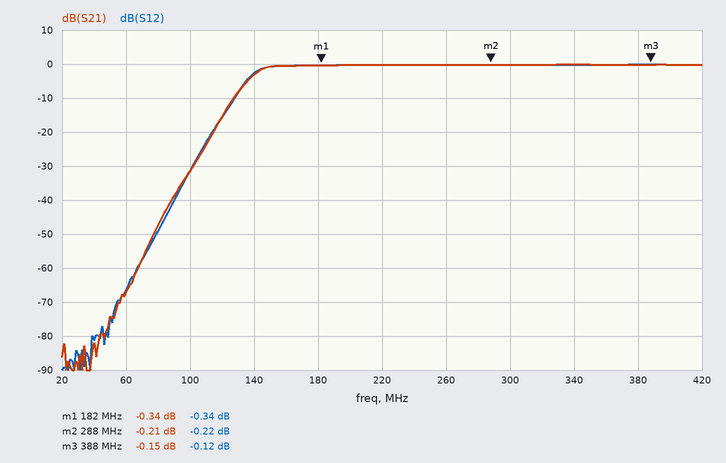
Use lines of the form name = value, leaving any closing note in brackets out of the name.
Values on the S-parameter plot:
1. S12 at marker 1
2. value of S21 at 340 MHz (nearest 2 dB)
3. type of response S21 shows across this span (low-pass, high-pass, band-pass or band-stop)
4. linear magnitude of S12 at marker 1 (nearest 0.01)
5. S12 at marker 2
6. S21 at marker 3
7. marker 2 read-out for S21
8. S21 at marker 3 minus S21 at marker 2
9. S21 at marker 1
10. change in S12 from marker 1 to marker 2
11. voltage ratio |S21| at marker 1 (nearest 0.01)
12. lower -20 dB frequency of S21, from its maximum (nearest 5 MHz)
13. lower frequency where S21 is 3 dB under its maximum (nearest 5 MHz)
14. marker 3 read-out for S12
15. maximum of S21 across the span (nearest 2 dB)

S12 at marker 1 = -0.34 dB
value of S21 at 340 MHz = 0 dB
type of response S21 shows across this span = high-pass
linear magnitude of S12 at marker 1 = 0.96
S12 at marker 2 = -0.22 dB
S21 at marker 3 = -0.15 dB
marker 2 read-out for S21 = -0.21 dB
S21 at marker 3 minus S21 at marker 2 = 0.06 dB
S21 at marker 1 = -0.34 dB
change in S12 from marker 1 to marker 2 = 0.12 dB
voltage ratio |S21| at marker 1 = 0.96
lower -20 dB frequency of S21, from its maximum = 115 MHz
lower frequency where S21 is 3 dB under its maximum = 140 MHz
marker 3 read-out for S12 = -0.12 dB
maximum of S21 across the span = 0 dB
